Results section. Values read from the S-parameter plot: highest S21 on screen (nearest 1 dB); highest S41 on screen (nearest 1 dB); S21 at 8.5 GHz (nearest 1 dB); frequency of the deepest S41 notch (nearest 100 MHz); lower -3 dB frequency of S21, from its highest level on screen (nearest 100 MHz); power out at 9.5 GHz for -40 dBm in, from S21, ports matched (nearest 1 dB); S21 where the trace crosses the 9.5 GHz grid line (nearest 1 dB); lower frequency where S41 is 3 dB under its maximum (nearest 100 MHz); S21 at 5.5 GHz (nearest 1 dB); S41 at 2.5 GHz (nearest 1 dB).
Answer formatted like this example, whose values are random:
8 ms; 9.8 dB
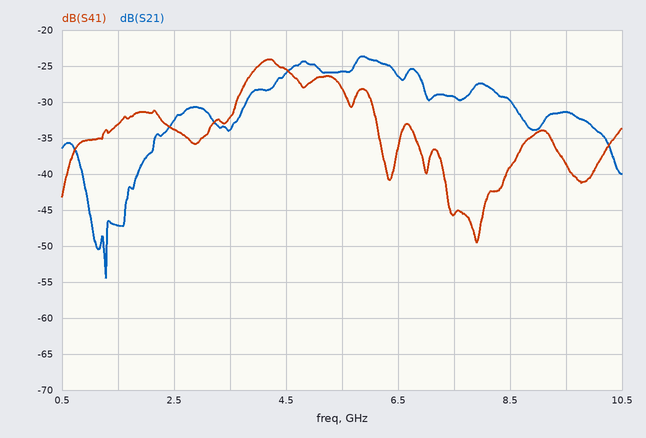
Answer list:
-24 dB; -24 dB; -30 dB; 7.9 GHz; 4.4 GHz; -71 dBm; -31 dB; 3.8 GHz; -26 dB; -34 dB
